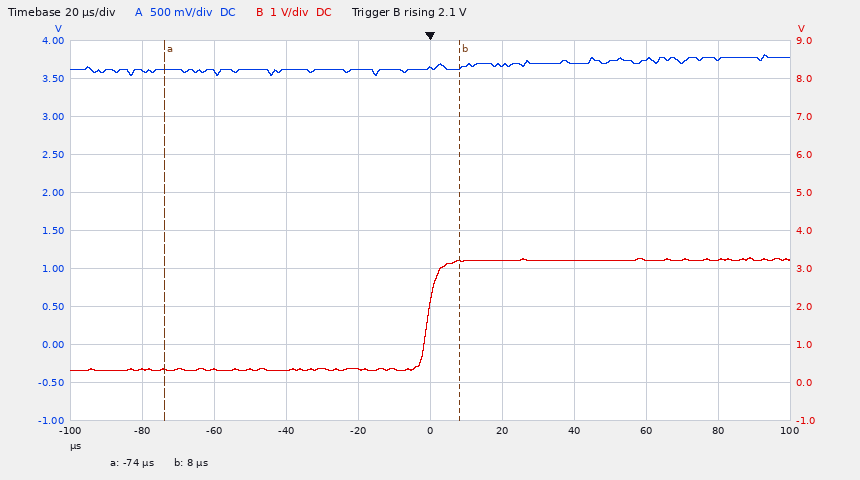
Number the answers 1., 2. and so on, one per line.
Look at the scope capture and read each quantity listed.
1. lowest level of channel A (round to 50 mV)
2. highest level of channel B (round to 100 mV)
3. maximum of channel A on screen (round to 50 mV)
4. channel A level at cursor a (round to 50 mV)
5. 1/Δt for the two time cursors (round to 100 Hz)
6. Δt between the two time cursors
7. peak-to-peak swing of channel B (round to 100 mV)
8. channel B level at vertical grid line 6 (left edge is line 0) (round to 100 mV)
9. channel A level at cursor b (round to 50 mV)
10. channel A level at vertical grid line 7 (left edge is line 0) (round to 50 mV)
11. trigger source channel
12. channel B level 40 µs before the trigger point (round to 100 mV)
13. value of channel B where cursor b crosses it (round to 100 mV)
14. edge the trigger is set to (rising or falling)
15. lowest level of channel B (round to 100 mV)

1. 3.55 V
2. 3.3 V
3. 3.80 V
4. 3.60 V
5. 12.2 kHz
6. 82 µs
7. 3.0 V
8. 3.2 V
9. 3.65 V
10. 3.70 V
11. channel B
12. 300 mV
13. 3.2 V
14. rising
15. 300 mV
